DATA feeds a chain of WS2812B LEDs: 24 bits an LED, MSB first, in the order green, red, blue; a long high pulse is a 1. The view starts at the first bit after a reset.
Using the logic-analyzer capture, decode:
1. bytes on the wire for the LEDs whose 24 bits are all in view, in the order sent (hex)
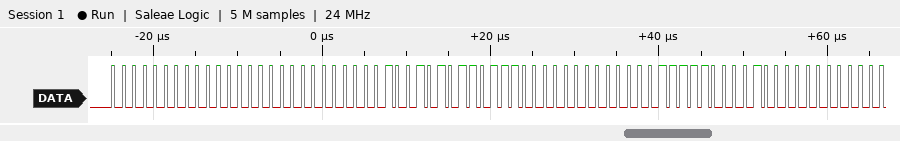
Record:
00 00 00 25 6E 00 0F 84 00
